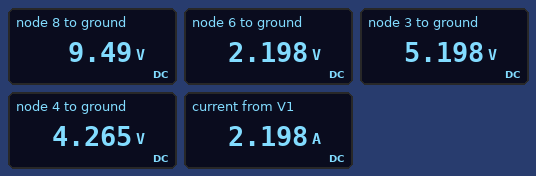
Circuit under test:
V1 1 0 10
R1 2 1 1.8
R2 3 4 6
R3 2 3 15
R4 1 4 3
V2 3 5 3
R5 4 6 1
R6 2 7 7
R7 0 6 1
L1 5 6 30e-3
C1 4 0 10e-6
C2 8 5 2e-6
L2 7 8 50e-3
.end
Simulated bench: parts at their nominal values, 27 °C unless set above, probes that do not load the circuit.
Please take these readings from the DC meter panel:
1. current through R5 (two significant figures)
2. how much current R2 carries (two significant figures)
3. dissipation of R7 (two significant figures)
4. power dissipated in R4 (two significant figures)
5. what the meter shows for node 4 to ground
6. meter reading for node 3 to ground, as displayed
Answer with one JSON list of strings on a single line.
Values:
["2.1 A", "160 mA", "4.8 W", "11 W", "4.265 V", "5.198 V"]
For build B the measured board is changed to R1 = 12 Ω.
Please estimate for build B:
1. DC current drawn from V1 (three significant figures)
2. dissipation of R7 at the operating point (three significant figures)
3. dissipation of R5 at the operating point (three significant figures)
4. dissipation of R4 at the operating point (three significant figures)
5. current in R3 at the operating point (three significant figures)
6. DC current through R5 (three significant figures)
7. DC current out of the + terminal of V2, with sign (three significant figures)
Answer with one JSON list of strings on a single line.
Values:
["2.11 A", "4.47 W", "4.35 W", "11.2 W", "181 mA", "2.09 A", "-28.6 mA"]
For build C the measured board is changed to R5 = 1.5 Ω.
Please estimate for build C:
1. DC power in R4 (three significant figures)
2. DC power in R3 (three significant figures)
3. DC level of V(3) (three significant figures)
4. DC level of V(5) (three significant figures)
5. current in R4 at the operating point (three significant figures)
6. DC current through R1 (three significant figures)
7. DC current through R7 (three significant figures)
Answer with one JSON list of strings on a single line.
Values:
["9.20 W", "1.30 W", "5.05 V", "2.05 V", "1.75 A", "295 mA", "2.05 A"]
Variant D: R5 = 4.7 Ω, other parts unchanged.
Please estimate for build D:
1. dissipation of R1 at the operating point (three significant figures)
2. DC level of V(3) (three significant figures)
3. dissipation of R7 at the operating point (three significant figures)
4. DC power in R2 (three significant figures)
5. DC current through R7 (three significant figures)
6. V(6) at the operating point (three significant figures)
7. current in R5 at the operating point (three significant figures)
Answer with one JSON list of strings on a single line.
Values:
["187 mW", "4.58 V", "2.50 W", "447 mW", "1.58 A", "1.58 V", "987 mA"]
